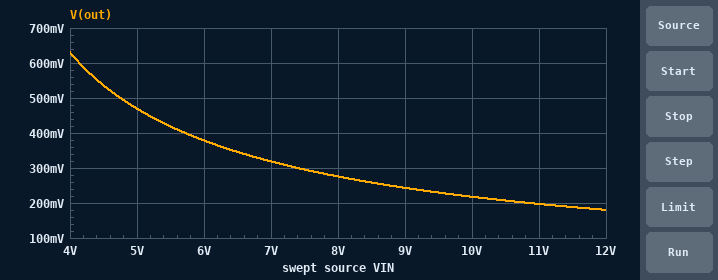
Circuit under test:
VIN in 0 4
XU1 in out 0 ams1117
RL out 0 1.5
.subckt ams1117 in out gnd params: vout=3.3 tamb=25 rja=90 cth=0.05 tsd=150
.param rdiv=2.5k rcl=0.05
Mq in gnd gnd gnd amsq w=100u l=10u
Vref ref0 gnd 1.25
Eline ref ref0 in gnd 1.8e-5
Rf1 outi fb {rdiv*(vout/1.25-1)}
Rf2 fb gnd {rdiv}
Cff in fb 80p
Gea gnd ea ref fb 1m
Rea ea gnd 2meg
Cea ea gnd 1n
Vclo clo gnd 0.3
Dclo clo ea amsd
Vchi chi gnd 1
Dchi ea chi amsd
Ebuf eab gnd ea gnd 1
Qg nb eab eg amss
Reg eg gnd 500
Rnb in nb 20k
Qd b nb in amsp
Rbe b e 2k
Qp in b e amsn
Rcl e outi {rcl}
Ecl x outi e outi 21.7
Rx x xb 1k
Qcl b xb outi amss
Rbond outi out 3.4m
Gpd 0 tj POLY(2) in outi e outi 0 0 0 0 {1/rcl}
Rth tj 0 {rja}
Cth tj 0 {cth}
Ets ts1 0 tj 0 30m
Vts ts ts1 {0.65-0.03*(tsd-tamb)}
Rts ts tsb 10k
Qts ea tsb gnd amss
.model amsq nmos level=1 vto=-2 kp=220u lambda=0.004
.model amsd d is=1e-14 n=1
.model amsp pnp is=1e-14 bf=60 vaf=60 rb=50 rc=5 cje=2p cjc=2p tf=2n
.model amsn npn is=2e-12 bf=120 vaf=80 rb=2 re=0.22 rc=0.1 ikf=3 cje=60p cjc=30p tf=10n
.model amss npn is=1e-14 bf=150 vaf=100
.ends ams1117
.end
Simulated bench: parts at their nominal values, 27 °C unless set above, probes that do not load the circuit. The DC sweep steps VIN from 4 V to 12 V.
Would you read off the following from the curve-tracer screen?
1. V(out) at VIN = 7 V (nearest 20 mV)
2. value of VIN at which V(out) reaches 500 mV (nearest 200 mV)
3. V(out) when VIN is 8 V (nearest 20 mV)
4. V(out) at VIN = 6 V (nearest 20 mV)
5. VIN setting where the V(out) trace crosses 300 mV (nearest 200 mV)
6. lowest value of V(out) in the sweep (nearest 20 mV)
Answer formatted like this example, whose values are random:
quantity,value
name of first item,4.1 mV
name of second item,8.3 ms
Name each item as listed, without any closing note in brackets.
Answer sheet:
quantity,value
V(out) at VIN = 7 V,320 mV
value of VIN at which V(out) reaches 500 mV,4.8 V
V(out) when VIN is 8 V,280 mV
V(out) at VIN = 6 V,380 mV
VIN setting where the V(out) trace crosses 300 mV,7.4 V
lowest value of V(out) in the sweep,180 mV
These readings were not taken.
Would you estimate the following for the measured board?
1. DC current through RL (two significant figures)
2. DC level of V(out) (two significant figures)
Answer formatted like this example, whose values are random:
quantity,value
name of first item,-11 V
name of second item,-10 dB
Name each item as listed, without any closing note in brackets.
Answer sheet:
quantity,value
DC current through RL,420 mA
DC level of V(out),630 mV
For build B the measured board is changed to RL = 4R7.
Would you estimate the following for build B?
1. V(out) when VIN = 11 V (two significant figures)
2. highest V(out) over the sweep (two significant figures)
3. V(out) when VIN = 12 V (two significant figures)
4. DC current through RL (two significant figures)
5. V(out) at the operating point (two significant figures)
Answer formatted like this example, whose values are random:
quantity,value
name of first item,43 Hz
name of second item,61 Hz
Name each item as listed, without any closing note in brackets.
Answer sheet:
quantity,value
V(out) when VIN = 11 V,640 mV
highest V(out) over the sweep,3.3 V
V(out) when VIN = 12 V,580 mV
DC current through RL,640 mA
V(out) at the operating point,3.0 V
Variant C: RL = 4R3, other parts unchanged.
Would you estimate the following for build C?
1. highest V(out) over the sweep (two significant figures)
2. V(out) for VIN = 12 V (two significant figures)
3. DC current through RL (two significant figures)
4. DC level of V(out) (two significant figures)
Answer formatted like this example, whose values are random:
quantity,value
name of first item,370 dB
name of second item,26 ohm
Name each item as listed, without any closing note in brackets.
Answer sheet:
quantity,value
highest V(out) over the sweep,3.3 V
V(out) for VIN = 12 V,530 mV
DC current through RL,690 mA
DC level of V(out),3.0 V
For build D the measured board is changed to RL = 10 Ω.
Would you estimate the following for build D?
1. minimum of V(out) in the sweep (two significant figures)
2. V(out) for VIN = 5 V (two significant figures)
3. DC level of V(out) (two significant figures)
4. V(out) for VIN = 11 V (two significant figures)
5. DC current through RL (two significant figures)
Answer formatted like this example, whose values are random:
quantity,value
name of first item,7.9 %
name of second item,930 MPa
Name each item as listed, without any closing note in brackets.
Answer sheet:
quantity,value
minimum of V(out) in the sweep,1.3 V
V(out) for VIN = 5 V,3.3 V
DC level of V(out),3.2 V
V(out) for VIN = 11 V,1.5 V
DC current through RL,320 mA
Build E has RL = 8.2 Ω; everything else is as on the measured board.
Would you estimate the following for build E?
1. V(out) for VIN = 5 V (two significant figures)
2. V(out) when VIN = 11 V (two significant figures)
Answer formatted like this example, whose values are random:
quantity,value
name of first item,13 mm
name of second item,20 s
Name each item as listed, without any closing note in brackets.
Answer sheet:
quantity,value
V(out) for VIN = 5 V,3.3 V
V(out) when VIN = 11 V,1.2 V
